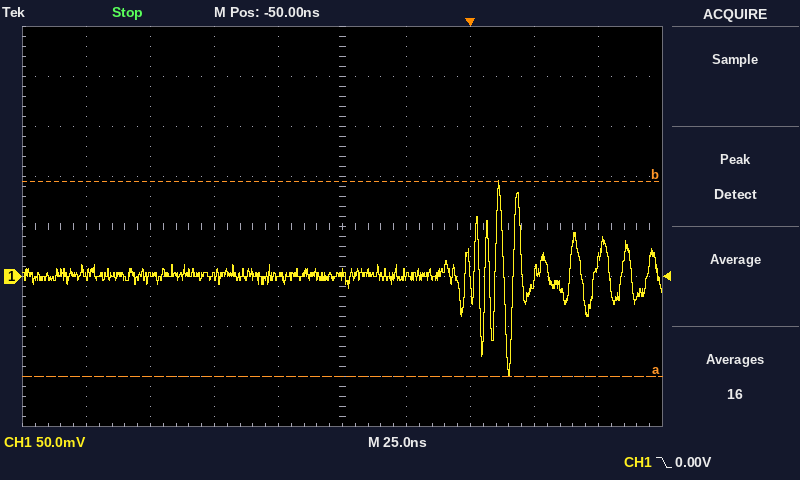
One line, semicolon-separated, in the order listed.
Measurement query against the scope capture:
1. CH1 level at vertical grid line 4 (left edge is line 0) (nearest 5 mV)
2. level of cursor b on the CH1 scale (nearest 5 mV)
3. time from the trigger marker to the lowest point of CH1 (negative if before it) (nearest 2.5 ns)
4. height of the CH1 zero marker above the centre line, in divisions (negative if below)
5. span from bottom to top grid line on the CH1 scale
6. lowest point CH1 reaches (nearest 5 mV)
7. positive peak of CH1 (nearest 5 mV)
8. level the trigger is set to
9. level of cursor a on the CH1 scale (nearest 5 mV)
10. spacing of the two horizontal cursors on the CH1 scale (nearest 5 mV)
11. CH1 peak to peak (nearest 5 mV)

0 mV; 95 mV; +15.0 ns; -1.0 div; 400 mV; -100 mV; 95 mV; 0.00 V; -100 mV; 195 mV; 195 mV
